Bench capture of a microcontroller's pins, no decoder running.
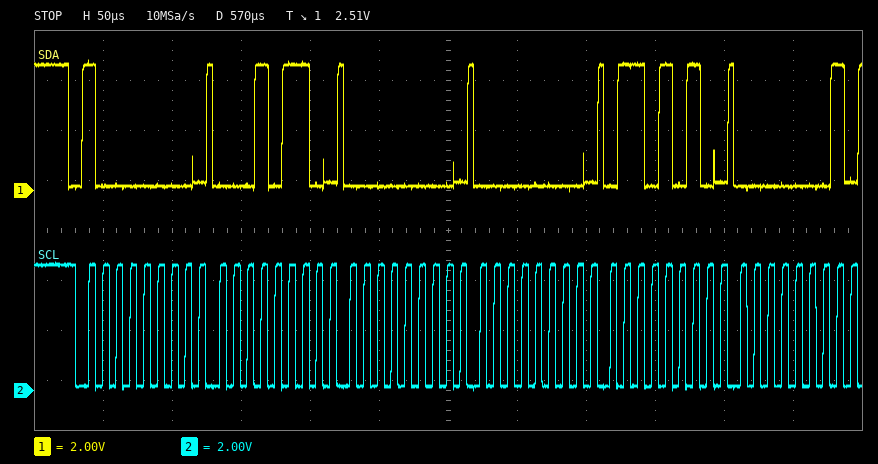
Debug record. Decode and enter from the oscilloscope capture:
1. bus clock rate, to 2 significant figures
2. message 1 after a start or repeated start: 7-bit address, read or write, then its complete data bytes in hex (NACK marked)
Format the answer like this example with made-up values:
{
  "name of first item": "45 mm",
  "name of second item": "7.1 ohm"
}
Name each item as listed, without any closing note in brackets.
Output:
{
  "bus clock rate, to 2 significant figures": "100 kHz",
  "message 1 after a start or repeated start: 7-bit address, read or write, then its complete data bytes in hex": "0x40 write: 16 00 00 6A 01"
}
